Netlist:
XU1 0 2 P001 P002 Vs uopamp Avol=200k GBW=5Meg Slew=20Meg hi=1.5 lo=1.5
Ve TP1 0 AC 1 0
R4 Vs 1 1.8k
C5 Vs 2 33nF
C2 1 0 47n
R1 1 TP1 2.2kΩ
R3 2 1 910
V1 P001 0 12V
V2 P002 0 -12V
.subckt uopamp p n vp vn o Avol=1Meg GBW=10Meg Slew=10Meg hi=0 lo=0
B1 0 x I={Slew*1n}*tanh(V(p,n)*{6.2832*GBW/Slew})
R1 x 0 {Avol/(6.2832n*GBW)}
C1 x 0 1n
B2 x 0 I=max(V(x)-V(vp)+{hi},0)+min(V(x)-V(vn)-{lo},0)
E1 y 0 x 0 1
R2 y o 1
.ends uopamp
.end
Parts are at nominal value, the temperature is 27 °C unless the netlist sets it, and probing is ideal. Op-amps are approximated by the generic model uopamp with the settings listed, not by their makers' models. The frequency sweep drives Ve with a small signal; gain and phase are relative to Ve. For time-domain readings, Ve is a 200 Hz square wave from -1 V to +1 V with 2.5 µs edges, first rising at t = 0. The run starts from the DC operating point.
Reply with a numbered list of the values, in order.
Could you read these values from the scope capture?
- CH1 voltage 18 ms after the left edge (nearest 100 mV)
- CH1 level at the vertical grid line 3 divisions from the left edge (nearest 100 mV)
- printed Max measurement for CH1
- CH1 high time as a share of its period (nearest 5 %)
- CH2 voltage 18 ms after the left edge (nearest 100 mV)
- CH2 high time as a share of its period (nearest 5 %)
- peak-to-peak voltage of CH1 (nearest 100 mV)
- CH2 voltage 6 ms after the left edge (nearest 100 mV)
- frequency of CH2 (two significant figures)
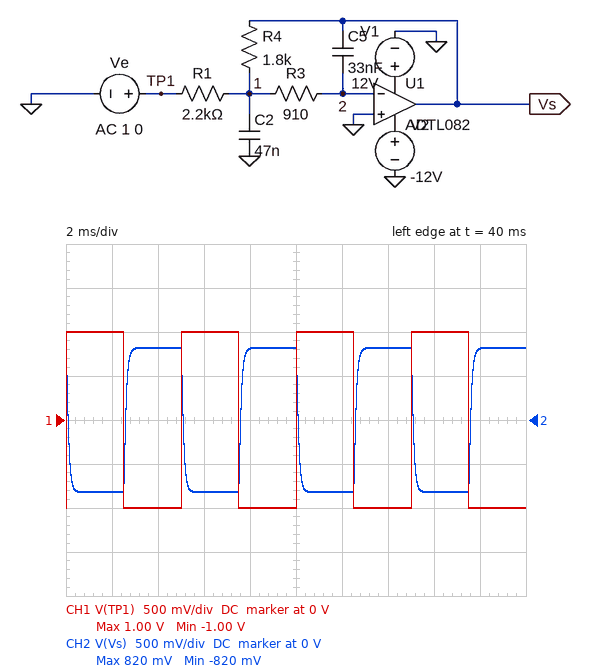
1. -1.0 V
2. 1.0 V
3. 1.00 V
4. 50 %
5. 800 mV
6. 50 %
7. 2.0 V
8. -800 mV
9. 200 Hz
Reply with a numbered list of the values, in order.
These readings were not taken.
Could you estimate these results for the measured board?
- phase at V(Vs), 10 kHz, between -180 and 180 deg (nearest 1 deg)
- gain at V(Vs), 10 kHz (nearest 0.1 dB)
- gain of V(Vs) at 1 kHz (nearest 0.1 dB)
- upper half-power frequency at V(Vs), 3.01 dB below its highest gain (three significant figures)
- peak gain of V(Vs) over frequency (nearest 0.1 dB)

1. 38 deg
2. -23.0 dB
3. -3.0 dB
4. 1.71 kHz
5. -1.7 dB
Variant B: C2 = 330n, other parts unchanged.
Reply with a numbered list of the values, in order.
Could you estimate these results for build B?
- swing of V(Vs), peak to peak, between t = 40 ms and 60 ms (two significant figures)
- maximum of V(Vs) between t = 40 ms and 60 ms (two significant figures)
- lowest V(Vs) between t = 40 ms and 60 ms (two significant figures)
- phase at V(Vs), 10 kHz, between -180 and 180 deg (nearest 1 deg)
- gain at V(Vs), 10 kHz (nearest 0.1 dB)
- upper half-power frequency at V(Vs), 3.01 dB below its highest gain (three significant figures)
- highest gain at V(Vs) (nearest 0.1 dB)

1. 2.4 V
2. 1.2 V
3. -1.2 V
4. 6 deg
5. -38.6 dB
6. 1.41 kHz
7. 0.5 dB
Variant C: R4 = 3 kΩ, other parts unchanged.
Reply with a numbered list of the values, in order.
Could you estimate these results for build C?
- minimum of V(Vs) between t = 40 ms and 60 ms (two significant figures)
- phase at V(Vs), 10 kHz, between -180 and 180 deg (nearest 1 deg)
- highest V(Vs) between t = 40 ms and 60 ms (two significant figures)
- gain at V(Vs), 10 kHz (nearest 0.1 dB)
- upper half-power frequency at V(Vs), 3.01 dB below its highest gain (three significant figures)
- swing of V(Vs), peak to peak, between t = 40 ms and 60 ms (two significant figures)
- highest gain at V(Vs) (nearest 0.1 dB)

1. -1.4 V
2. 34 deg
3. 1.4 V
4. -22.9 dB
5. 1.09 kHz
6. 2.7 V
7. 2.7 dB
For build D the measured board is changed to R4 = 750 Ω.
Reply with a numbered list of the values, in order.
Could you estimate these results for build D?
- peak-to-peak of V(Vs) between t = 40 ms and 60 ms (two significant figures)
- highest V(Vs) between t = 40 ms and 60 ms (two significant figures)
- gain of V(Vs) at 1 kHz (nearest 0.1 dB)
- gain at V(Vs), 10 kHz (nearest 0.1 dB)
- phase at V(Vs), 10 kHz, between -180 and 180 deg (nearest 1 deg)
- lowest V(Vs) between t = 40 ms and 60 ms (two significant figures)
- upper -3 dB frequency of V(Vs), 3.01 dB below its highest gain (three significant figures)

1. 680 mV
2. 340 mV
3. -9.7 dB
4. -23.6 dB
5. 52 deg
6. -340 mV
7. 3.15 kHz
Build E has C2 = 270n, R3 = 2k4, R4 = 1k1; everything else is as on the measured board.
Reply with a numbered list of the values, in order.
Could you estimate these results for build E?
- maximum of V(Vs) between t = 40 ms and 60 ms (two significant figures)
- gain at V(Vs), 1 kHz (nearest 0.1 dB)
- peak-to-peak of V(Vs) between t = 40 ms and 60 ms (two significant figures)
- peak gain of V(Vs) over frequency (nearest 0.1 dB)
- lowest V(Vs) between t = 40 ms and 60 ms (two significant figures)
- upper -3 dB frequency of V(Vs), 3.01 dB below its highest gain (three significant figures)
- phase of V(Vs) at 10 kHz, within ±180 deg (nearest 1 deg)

1. 660 mV
2. -5.8 dB
3. 1.3 V
4. -4.8 dB
5. -660 mV
6. 1.21 kHz
7. 6 deg
